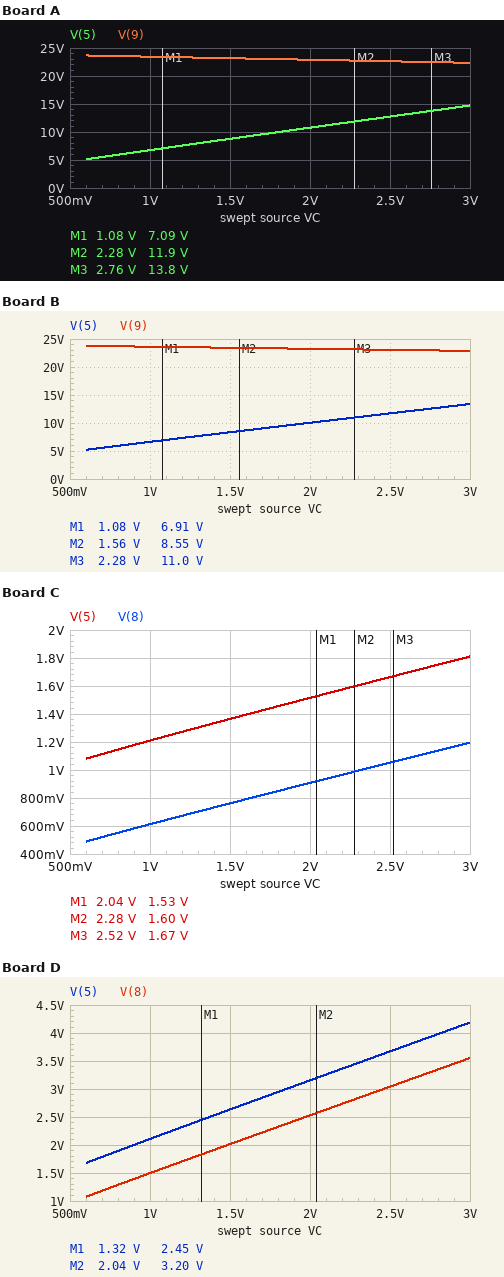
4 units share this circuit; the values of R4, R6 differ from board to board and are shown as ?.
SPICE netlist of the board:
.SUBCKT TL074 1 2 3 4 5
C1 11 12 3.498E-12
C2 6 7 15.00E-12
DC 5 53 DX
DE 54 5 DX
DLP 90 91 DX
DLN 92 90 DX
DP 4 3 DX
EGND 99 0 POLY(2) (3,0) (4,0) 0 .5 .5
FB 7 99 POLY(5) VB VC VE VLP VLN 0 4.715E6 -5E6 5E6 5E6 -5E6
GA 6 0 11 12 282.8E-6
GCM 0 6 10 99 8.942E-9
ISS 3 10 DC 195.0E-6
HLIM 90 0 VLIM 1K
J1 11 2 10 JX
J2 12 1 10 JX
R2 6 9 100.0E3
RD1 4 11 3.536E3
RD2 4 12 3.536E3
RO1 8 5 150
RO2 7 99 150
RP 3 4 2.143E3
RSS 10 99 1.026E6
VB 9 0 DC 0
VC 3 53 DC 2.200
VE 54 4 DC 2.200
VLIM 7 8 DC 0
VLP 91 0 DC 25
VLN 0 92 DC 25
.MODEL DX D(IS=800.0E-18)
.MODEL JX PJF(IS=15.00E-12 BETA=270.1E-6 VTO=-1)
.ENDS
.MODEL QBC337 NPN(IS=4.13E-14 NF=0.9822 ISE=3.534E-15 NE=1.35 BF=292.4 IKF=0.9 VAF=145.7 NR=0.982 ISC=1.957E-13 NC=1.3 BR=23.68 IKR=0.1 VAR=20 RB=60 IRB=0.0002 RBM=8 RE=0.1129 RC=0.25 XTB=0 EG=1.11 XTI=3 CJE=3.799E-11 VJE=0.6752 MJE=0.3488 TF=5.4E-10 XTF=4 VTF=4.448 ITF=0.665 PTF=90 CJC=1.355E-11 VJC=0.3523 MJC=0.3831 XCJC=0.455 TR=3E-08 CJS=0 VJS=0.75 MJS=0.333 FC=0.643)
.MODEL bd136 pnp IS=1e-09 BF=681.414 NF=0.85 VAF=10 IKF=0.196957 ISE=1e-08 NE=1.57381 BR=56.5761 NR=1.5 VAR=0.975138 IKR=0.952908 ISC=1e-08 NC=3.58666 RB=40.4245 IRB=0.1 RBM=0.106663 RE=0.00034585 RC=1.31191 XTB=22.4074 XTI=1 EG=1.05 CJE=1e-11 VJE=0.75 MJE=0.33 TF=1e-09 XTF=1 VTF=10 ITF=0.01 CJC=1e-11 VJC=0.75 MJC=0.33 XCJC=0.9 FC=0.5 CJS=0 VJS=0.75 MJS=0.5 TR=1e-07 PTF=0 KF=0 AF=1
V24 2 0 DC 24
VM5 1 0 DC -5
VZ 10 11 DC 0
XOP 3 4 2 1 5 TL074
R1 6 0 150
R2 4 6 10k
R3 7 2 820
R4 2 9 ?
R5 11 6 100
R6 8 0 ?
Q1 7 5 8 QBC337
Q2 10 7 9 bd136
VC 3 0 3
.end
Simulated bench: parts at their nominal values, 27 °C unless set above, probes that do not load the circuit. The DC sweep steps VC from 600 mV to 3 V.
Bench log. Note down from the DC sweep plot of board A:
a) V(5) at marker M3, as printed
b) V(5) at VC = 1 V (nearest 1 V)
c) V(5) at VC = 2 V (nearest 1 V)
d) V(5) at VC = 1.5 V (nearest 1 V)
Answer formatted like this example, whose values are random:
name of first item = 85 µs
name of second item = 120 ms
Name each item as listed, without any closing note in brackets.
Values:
V(5) at marker M3, as printed = 13.8 V
V(5) at VC = 1 V = 7 V
V(5) at VC = 2 V = 11 V
V(5) at VC = 1.5 V = 9 V
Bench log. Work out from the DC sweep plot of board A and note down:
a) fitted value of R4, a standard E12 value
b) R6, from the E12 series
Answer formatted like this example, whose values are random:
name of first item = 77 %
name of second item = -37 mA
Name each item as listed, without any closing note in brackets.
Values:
fitted value of R4, a standard E12 value = 82 Ω
R6, from the E12 series = 5.6 kΩ
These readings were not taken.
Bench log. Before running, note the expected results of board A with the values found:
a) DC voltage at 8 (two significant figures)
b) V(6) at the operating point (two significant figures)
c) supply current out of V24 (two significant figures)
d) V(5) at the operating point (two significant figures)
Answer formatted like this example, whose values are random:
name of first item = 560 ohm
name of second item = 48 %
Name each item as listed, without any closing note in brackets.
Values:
DC voltage at 8 = 14 V
V(6) at the operating point = 3.0 V
supply current out of V24 = 36 mA
V(5) at the operating point = 15 V
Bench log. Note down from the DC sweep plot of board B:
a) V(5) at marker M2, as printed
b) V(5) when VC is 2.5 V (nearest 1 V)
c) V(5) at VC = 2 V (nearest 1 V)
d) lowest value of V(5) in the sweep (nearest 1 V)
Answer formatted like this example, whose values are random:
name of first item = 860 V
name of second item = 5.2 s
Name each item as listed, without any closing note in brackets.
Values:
V(5) at marker M2, as printed = 8.55 V
V(5) when VC is 2.5 V = 12 V
V(5) at VC = 2 V = 10 V
lowest value of V(5) in the sweep = 5 V
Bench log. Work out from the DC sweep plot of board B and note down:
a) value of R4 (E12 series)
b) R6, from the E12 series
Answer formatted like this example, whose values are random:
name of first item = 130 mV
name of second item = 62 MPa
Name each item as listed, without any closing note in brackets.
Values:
value of R4 = 56 Ω
R6, from the E12 series = 6.8 kΩ
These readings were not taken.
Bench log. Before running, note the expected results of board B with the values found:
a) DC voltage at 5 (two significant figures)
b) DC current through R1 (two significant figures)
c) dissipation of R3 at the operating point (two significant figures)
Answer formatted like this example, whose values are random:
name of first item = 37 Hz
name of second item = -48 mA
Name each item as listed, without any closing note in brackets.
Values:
DC voltage at 5 = 13 V
DC current through R1 = 20 mA
dissipation of R3 at the operating point = 2.7 mW
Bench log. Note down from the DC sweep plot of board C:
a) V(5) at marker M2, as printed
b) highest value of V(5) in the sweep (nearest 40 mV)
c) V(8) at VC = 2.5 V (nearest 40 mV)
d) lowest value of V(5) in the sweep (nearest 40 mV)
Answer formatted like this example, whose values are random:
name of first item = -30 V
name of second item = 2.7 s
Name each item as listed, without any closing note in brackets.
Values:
V(5) at marker M2, as printed = 1.60 V
highest value of V(5) in the sweep = 1.80 V
V(8) at VC = 2.5 V = 1.04 V
lowest value of V(5) in the sweep = 1.08 V
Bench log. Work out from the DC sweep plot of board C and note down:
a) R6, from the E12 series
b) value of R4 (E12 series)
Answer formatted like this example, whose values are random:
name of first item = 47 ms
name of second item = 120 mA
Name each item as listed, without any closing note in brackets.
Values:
R6, from the E12 series = 820 Ω
value of R4 = 39 Ω
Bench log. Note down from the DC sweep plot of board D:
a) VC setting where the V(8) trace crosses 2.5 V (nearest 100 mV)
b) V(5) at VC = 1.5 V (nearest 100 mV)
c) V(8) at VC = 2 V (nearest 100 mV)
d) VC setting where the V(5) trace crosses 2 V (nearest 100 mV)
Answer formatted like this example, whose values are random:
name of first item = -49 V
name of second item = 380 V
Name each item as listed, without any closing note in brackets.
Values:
VC setting where the V(8) trace crosses 2.5 V = 2.0 V
V(5) at VC = 1.5 V = 2.6 V
V(8) at VC = 2 V = 2.5 V
VC setting where the V(5) trace crosses 2 V = 900 mV
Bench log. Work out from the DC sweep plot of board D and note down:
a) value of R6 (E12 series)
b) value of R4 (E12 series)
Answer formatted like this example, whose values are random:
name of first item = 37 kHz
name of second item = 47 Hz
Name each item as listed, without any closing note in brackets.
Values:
value of R6 = 1.2 kΩ
value of R4 = 100 Ω
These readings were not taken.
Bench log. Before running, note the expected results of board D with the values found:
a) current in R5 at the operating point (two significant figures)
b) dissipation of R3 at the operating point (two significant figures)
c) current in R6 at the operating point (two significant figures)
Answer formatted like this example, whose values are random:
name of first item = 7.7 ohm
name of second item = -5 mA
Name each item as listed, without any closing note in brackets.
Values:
current in R5 at the operating point = 20 mA
dissipation of R3 at the operating point = 6.8 mW
current in R6 at the operating point = 3.0 mA
